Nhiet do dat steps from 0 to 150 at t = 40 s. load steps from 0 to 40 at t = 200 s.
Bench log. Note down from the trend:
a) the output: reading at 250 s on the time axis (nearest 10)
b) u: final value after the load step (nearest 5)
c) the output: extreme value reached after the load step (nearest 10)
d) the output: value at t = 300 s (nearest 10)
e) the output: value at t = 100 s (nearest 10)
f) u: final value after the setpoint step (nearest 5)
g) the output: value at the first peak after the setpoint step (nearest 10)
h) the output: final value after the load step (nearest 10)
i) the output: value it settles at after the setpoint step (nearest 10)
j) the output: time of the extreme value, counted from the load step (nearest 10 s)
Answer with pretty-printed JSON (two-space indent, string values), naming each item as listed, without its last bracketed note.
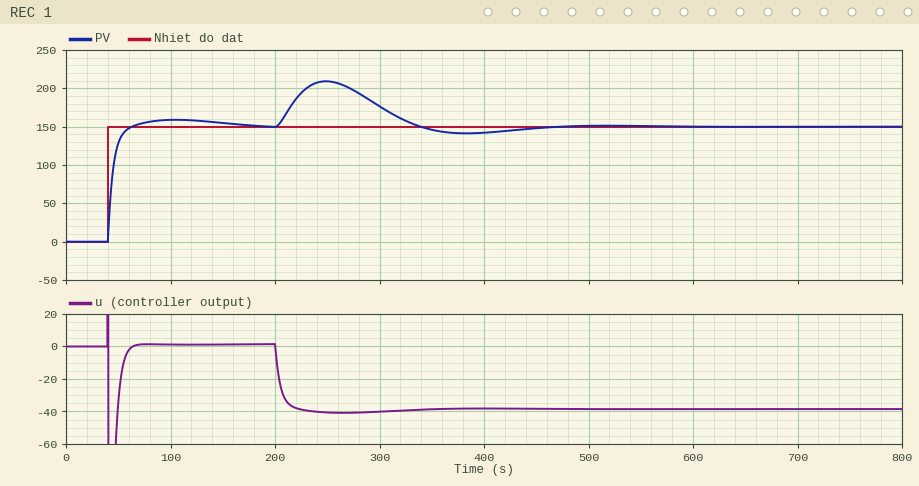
{
  "the output: reading at 250 s on the time axis": "210",
  "u: final value after the load step": "-40",
  "the output: extreme value reached after the load step": "210",
  "the output: value at t = 300 s": "180",
  "the output: value at t = 100 s": "160",
  "u: final value after the setpoint step": "0",
  "the output: value at the first peak after the setpoint step": "160",
  "the output: final value after the load step": "150",
  "the output: value it settles at after the setpoint step": "150",
  "the output: time of the extreme value, counted from the load step": "50 s"
}
